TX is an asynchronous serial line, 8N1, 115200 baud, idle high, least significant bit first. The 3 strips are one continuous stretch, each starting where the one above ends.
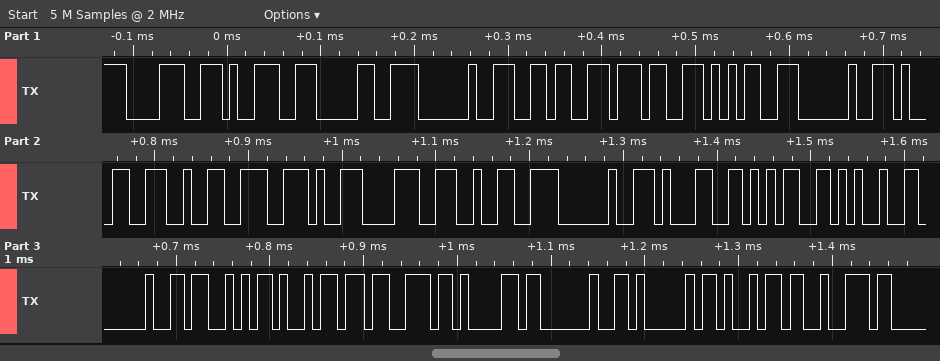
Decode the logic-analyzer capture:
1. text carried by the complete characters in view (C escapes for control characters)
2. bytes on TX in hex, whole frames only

"890 675 12.82 15% Sisa Air"
38 39 30 20 36 37 35 20 31 32 2E 38 32 20 31 35 25 20 53 69 73 61 20 41 69 72
